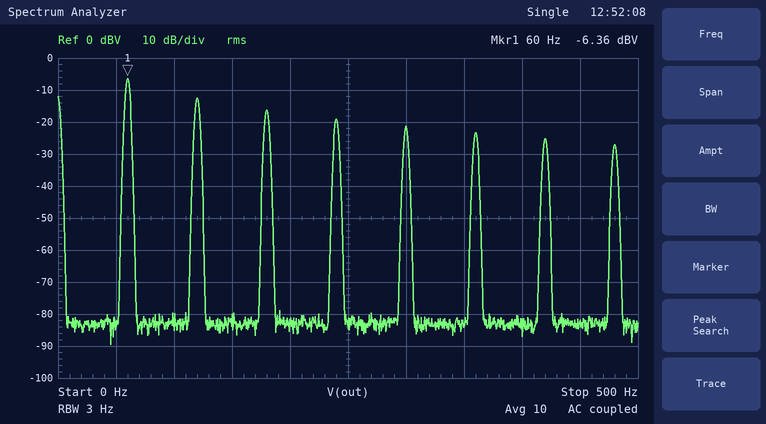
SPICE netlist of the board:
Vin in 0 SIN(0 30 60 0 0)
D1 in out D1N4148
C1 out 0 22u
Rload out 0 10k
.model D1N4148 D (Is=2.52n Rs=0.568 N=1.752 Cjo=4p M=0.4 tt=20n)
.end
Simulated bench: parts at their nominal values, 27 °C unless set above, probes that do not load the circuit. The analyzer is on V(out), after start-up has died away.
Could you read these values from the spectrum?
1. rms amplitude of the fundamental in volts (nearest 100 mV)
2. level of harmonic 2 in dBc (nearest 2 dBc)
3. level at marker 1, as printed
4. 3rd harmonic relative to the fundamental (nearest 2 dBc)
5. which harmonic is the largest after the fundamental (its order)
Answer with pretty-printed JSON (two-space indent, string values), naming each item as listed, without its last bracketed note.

{
  "rms amplitude of the fundamental in volts": "500 mV",
  "level of harmonic 2 in dBc": "-6 dBc",
  "level at marker 1, as printed": "-6.36 dBV",
  "3rd harmonic relative to the fundamental": "-10 dBc",
  "which harmonic is the largest after the fundamental": "2"
}
